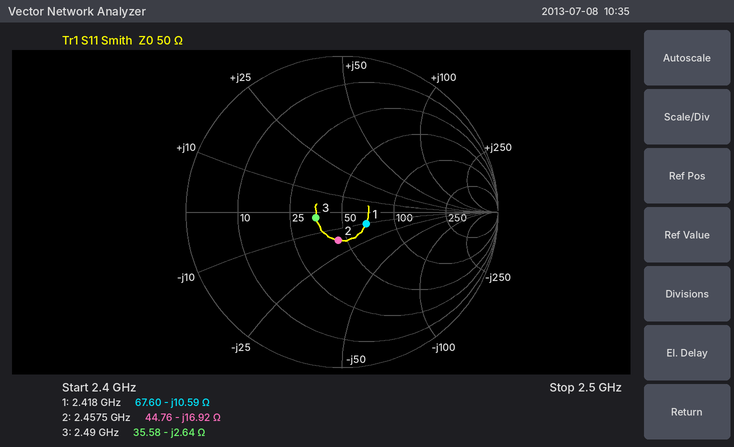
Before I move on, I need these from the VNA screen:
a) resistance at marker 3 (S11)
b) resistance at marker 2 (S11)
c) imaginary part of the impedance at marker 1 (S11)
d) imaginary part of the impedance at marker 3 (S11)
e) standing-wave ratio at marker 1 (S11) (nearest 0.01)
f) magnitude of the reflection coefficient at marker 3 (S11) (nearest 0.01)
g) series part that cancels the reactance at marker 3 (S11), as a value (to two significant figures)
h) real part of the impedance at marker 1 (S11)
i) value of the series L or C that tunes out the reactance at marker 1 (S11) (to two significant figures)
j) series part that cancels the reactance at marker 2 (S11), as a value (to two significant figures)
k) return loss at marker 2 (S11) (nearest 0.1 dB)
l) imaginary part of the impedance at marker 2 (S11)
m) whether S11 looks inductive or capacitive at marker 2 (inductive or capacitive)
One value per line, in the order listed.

35.58 Ω
44.76 Ω
-10.59 Ω
-2.64 Ω
1.42
0.17
170 pH
67.60 Ω
700 pH
1.1 nH
14.7 dB
-16.92 Ω
capacitive
